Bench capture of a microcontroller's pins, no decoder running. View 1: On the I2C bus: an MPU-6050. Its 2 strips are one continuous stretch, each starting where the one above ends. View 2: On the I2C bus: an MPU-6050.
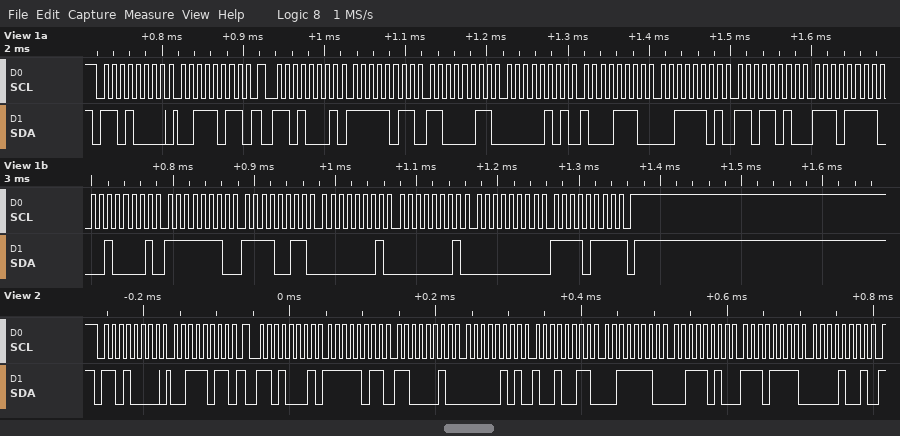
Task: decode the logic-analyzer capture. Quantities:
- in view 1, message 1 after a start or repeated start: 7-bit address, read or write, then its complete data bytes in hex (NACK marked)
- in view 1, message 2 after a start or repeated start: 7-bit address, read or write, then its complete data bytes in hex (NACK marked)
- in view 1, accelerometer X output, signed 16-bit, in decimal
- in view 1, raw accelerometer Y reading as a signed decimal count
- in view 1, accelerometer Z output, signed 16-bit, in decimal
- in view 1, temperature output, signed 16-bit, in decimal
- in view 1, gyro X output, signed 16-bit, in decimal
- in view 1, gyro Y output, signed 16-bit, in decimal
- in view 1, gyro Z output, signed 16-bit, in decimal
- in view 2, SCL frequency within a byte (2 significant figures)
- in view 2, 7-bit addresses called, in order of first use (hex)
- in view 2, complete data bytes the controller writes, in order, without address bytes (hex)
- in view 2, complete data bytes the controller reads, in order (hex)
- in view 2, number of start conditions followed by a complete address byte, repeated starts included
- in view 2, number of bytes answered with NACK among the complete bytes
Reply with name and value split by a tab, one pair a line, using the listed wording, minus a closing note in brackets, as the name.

in view 1, message 1 after a start or repeated start: 7-bit address, read or write, then its complete data bytes in hex	0x68 write: 3B
in view 1, message 2 after a start or repeated start: 7-bit address, read or write, then its complete data bytes in hex	0x68 read: FB C3 05 8E 3D DA EF 21 FE F3 01 01 00 F7 NACK
in view 1, accelerometer X output, signed 16-bit, in decimal	-1085
in view 1, raw accelerometer Y reading as a signed decimal count	1422
in view 1, accelerometer Z output, signed 16-bit, in decimal	15834
in view 1, temperature output, signed 16-bit, in decimal	-4319
in view 1, gyro X output, signed 16-bit, in decimal	-269
in view 1, gyro Y output, signed 16-bit, in decimal	257
in view 1, gyro Z output, signed 16-bit, in decimal	247
in view 2, SCL frequency within a byte	100 kHz
in view 2, 7-bit addresses called, in order of first use	0x68
in view 2, complete data bytes the controller writes, in order, without address bytes	3B
in view 2, complete data bytes the controller reads, in order	FB C2 05 93 3E 3A EF 09
in view 2, number of start conditions followed by a complete address byte, repeated starts included	2
in view 2, number of bytes answered with NACK among the complete bytes	0
